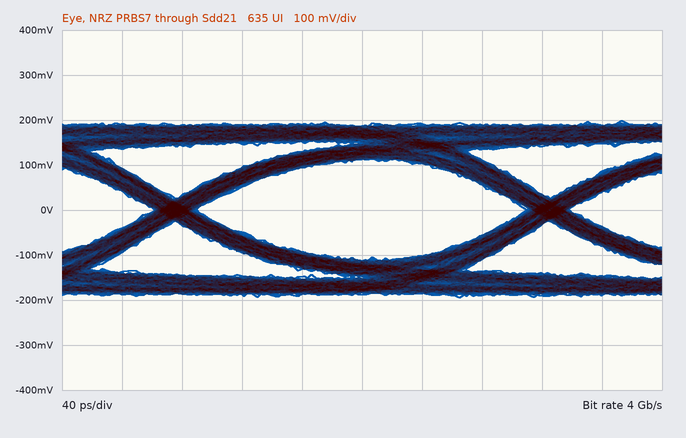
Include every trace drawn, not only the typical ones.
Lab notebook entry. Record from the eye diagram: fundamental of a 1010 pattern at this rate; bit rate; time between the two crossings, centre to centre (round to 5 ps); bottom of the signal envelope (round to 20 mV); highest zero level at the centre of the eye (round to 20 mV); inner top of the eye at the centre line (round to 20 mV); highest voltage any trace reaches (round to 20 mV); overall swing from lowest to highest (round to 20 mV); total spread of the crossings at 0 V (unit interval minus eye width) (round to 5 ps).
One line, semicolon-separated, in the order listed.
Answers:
2 GHz; 4 Gb/s; 250 ps; -200 mV; -120 mV; 120 mV; 200 mV; 400 mV; 30 ps
